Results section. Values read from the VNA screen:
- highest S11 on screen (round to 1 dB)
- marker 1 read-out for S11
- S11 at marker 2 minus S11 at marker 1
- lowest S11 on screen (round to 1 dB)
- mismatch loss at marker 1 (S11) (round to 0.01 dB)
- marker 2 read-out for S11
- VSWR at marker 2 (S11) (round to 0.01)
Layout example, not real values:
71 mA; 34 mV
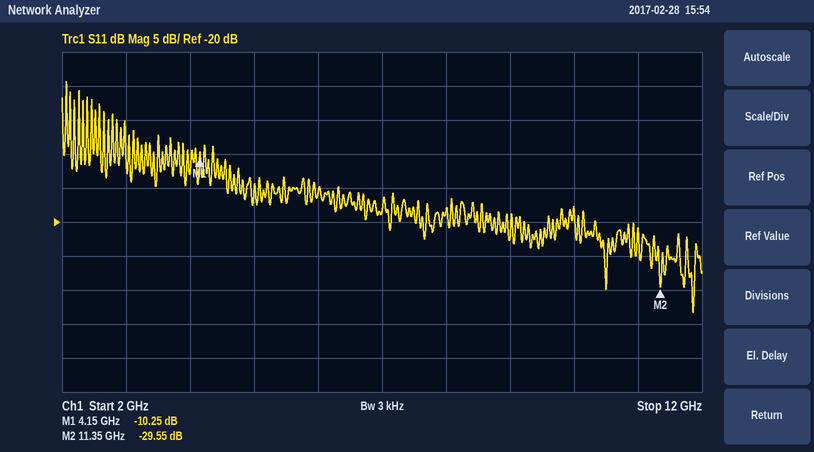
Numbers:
1 dB; -10.25 dB; -19.30 dB; -33 dB; 0.43 dB; -29.55 dB; 1.07
